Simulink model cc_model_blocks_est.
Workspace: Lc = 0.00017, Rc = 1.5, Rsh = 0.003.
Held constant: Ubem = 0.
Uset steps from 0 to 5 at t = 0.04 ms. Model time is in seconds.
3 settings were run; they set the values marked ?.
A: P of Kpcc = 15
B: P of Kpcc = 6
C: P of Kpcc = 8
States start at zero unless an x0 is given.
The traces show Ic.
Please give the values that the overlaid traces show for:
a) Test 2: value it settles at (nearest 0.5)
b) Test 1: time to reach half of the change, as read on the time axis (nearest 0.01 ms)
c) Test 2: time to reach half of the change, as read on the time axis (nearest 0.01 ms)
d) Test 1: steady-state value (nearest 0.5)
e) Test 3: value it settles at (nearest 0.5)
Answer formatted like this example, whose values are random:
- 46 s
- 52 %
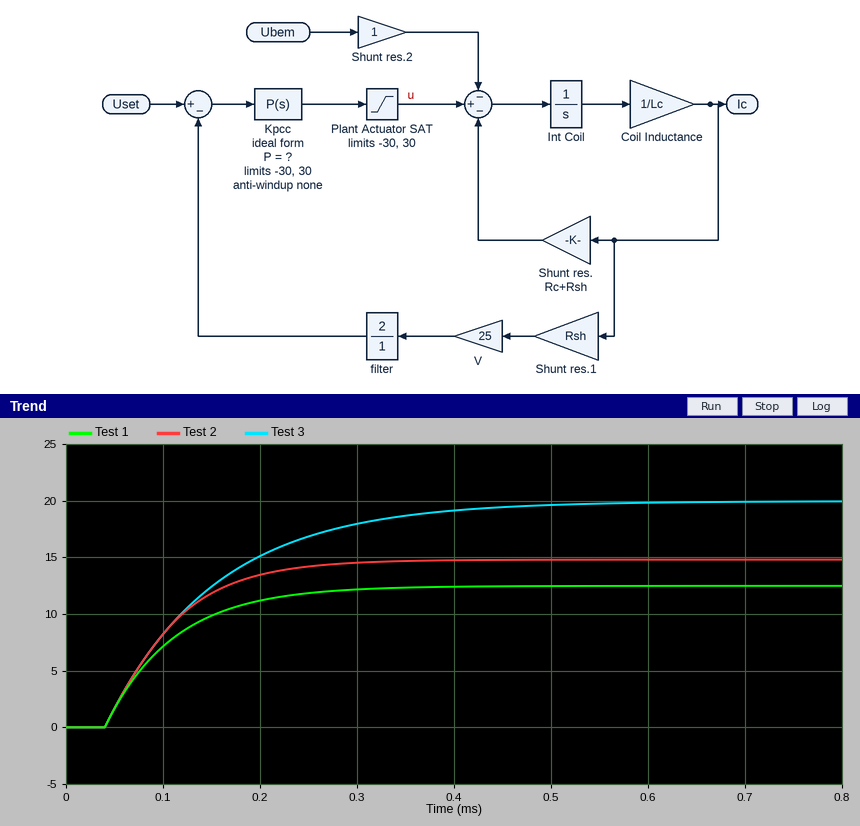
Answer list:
- 15.0
- 0.09 ms
- 0.09 ms
- 12.5
- 20.0
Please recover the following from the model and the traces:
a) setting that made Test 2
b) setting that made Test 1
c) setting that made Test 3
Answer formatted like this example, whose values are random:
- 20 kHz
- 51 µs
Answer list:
- C
- B
- A
